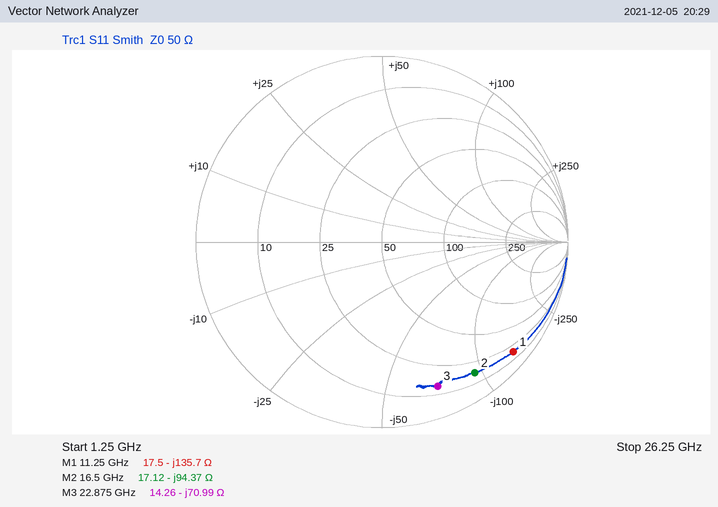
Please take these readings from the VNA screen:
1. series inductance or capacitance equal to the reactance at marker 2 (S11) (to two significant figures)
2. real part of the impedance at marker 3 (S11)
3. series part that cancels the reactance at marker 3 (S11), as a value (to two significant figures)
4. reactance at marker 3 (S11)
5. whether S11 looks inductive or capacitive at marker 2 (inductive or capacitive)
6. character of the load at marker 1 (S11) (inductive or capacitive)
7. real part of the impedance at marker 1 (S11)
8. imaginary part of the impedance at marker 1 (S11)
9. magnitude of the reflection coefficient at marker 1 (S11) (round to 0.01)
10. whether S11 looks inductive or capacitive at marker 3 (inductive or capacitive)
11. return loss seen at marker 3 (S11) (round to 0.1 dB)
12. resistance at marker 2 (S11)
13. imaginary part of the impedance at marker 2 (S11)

100 fF
14.26 Ω
490 pH
-70.99 Ω
capacitive
capacitive
17.5 Ω
-135.7 Ω
0.92
capacitive
1.6 dB
17.12 Ω
-94.37 Ω
